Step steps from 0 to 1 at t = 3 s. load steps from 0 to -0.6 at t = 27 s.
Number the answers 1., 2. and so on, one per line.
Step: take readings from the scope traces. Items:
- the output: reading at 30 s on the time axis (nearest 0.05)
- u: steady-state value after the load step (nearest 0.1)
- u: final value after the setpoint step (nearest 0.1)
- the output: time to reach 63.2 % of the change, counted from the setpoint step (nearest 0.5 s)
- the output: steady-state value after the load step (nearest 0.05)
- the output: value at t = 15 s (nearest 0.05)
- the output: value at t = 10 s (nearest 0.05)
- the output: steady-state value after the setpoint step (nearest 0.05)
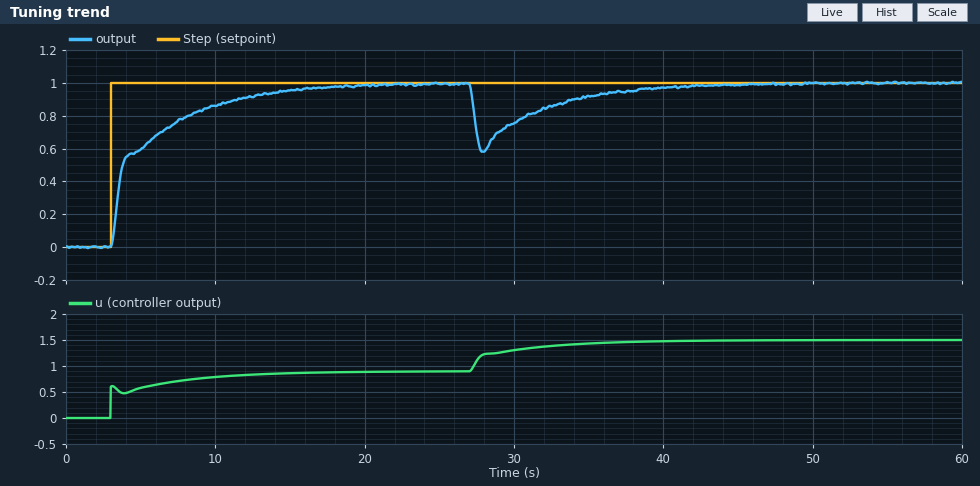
1. 0.75
2. 1.5
3. 0.9
4. 2.5 s
5. 1.00
6. 0.95
7. 0.85
8. 1.00
